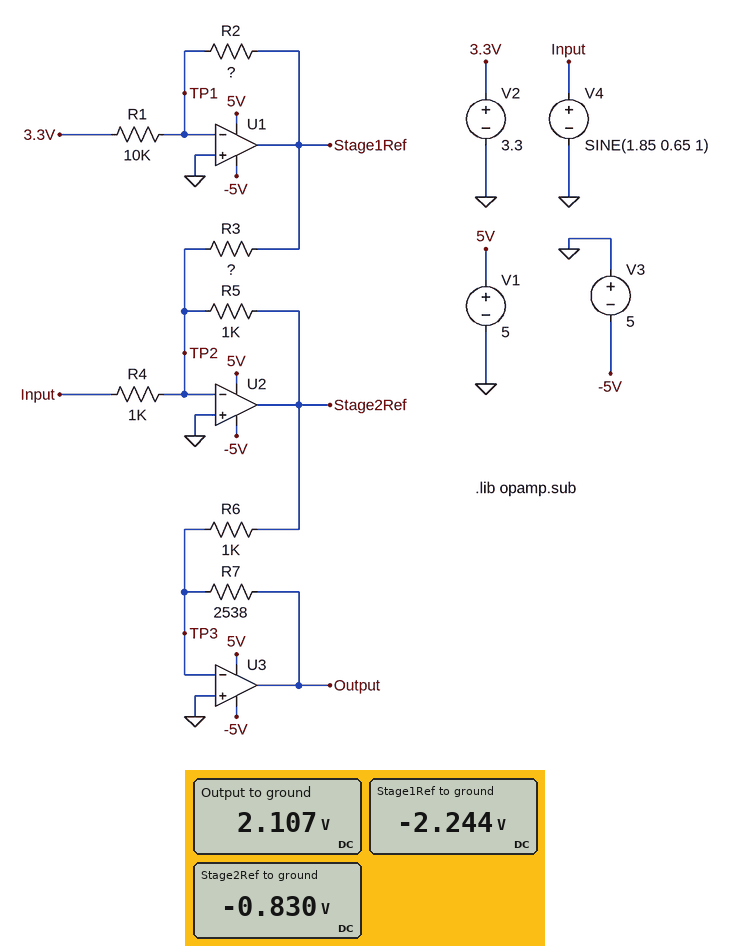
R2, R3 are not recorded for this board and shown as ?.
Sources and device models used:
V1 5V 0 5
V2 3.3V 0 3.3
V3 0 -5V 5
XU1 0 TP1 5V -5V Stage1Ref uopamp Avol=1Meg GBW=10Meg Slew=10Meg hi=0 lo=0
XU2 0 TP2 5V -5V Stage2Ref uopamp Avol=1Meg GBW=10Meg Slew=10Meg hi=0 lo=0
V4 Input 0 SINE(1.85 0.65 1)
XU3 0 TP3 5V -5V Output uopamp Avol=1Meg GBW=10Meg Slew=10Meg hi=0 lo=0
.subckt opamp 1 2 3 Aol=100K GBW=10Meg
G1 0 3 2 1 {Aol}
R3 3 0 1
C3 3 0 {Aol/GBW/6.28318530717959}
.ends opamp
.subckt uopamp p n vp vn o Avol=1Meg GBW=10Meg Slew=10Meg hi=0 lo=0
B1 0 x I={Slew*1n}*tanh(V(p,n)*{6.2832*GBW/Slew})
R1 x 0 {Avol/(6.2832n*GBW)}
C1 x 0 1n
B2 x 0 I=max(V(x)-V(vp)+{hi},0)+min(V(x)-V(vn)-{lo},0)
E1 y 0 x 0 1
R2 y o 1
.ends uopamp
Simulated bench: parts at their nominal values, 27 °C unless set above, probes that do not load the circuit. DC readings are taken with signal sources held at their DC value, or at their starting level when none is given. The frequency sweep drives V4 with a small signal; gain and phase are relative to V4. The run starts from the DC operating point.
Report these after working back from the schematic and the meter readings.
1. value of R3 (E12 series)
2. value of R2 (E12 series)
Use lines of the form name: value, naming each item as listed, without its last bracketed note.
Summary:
value of R3: 2.2 kΩ
value of R2: 6.8 kΩ
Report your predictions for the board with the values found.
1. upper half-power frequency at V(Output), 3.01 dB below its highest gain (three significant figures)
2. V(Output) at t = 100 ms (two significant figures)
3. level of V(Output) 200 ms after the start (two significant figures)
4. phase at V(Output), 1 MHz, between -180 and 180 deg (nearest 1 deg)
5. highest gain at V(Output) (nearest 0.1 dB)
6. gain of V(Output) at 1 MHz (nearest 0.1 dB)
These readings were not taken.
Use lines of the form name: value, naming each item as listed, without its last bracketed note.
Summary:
upper half-power frequency at V(Output), 3.01 dB below its highest gain: 2.13 MHz
V(Output) at t = 100 ms: 3.1 V
level of V(Output) 200 ms after the start: 3.7 V
phase at V(Output), 1 MHz, between -180 and 180 deg: -33 deg
highest gain at V(Output): 8.1 dB
gain of V(Output) at 1 MHz: 7.3 dB
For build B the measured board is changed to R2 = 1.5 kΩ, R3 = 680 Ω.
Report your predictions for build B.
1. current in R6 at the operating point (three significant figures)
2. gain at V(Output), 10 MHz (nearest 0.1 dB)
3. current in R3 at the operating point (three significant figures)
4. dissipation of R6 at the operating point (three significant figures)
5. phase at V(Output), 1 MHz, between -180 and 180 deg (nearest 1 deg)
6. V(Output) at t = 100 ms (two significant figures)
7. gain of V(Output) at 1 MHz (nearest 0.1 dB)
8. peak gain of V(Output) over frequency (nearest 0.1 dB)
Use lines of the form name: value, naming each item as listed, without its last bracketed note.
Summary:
current in R6 at the operating point: 1.12 mA
gain at V(Output), 10 MHz: -14.4 dB
current in R3 at the operating point: 728 µA
dissipation of R6 at the operating point: 1.26 mW
phase at V(Output), 1 MHz, between -180 and 180 deg: -39 deg
V(Output) at t = 100 ms: 3.8 V
gain of V(Output) at 1 MHz: 7.1 dB
peak gain of V(Output) over frequency: 8.1 dB
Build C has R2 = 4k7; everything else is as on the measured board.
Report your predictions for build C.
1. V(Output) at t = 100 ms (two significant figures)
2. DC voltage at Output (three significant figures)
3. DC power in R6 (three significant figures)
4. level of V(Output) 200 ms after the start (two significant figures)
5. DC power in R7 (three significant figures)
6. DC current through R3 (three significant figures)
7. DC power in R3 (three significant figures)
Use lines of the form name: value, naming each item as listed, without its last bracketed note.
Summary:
V(Output) at t = 100 ms: 3.9 V
DC voltage at Output: 2.91 V
DC power in R6: 1.31 mW
level of V(Output) 200 ms after the start: 4.5 V
DC power in R7: 3.33 mW
DC current through R3: 705 µA
DC power in R3: 1.09 mW
